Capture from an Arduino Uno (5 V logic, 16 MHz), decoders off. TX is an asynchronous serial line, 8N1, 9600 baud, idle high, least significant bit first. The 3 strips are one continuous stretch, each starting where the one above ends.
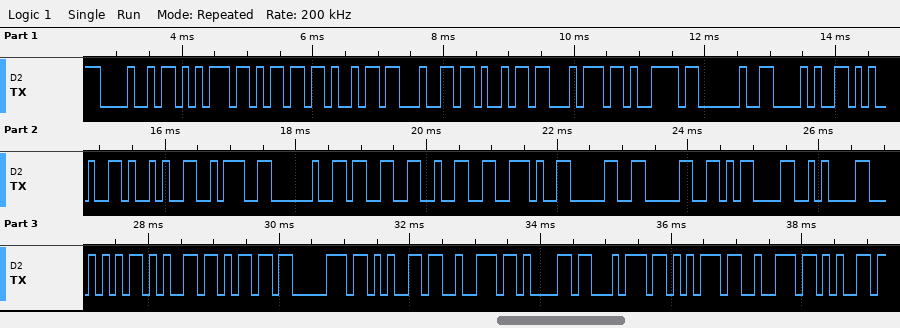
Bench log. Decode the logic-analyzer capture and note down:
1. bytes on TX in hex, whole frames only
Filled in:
48 75 6D 69 64 69 74 79 20 28 25 29 3A 20 33 32 2E 30 30 0D 0A 54 65 6D 70 65 72 61 74 75 72 65
